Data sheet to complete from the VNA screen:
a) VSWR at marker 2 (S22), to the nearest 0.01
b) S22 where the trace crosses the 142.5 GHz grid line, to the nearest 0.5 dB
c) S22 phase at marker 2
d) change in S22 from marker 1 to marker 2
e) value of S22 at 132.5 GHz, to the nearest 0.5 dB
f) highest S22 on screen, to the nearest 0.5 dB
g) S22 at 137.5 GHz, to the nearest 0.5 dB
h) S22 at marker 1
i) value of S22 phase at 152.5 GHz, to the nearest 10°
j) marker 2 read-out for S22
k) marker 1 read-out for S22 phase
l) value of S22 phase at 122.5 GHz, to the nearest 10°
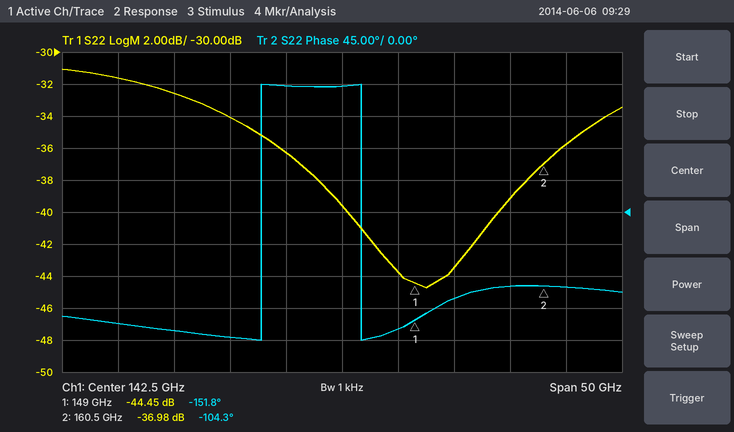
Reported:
1.03
-39.5 dB
-104.3°
7.47 dB
-34.0 dB
-31.0 dB
-36.5 dB
-44.45 dB
-120°
-36.98 dB
-151.8°
-160°
